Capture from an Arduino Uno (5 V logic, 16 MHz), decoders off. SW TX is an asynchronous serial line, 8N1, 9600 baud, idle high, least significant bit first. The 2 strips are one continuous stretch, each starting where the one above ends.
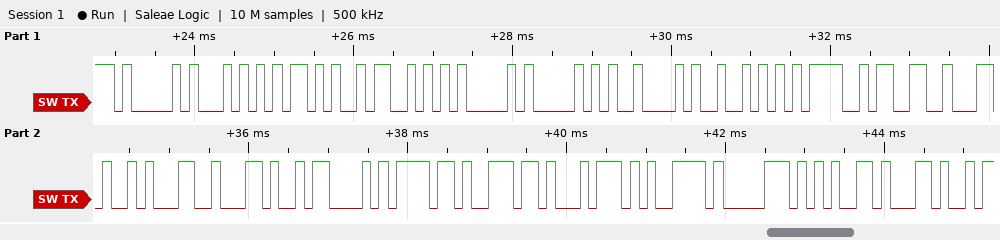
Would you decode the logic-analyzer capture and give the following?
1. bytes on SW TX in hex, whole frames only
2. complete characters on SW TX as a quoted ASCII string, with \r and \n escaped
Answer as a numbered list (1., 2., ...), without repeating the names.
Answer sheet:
1. 41 54 2B 53 41 50 42 52 3D 33 2C 31 2C 43 6F 6E 74 79 70 65 2C
2. "AT+SAPBR=3,1,Contype,"
